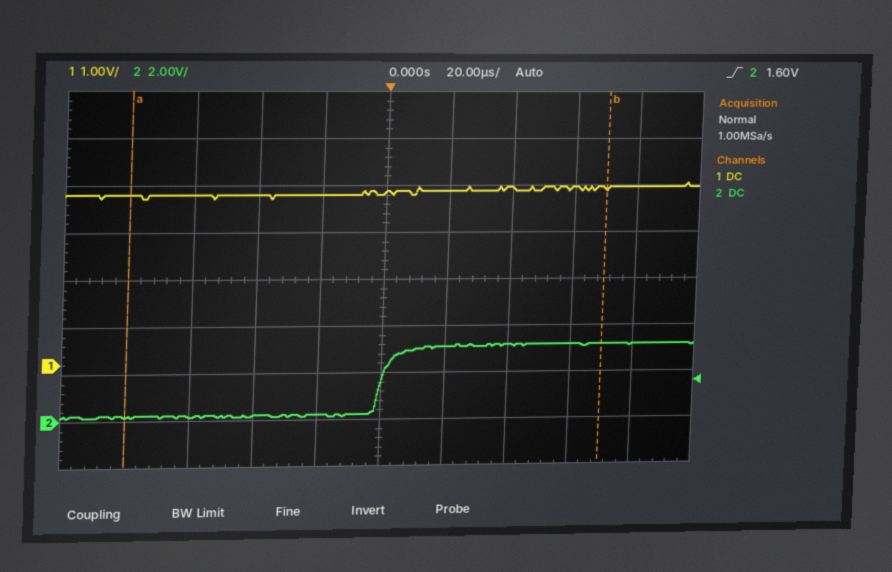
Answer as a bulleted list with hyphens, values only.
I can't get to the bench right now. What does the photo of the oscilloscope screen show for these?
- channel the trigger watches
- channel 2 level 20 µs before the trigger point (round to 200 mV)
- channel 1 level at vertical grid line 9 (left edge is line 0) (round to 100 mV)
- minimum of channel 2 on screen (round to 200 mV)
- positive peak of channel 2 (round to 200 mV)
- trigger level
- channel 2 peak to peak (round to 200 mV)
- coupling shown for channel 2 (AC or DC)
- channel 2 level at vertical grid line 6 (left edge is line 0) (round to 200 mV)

- channel 2
- 200 mV
- 3.8 V
- 200 mV
- 3.2 V
- 1.60 V
- 3.0 V
- DC
- 3.2 V
